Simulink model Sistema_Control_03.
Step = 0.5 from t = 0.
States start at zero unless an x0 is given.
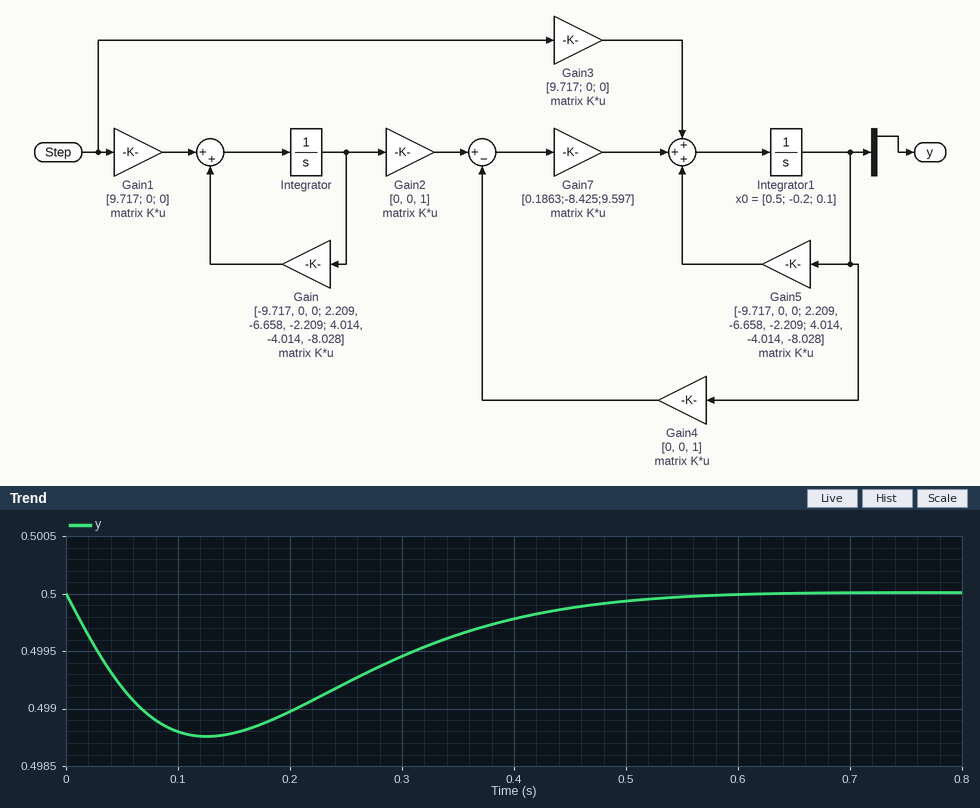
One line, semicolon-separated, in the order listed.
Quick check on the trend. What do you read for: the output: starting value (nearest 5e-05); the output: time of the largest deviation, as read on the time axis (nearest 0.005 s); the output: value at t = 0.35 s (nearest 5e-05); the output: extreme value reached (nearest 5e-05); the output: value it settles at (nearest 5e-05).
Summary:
0.50000; 0.125 s; 0.49965; 0.49875; 0.50000
